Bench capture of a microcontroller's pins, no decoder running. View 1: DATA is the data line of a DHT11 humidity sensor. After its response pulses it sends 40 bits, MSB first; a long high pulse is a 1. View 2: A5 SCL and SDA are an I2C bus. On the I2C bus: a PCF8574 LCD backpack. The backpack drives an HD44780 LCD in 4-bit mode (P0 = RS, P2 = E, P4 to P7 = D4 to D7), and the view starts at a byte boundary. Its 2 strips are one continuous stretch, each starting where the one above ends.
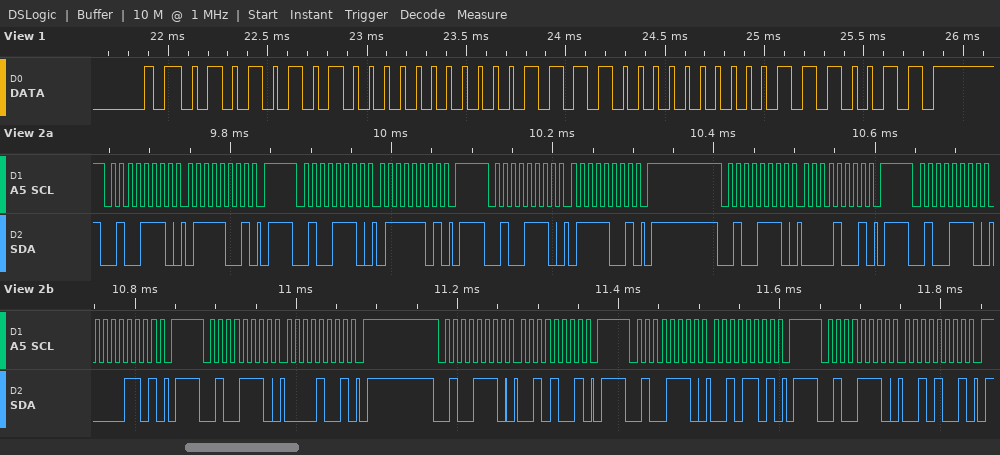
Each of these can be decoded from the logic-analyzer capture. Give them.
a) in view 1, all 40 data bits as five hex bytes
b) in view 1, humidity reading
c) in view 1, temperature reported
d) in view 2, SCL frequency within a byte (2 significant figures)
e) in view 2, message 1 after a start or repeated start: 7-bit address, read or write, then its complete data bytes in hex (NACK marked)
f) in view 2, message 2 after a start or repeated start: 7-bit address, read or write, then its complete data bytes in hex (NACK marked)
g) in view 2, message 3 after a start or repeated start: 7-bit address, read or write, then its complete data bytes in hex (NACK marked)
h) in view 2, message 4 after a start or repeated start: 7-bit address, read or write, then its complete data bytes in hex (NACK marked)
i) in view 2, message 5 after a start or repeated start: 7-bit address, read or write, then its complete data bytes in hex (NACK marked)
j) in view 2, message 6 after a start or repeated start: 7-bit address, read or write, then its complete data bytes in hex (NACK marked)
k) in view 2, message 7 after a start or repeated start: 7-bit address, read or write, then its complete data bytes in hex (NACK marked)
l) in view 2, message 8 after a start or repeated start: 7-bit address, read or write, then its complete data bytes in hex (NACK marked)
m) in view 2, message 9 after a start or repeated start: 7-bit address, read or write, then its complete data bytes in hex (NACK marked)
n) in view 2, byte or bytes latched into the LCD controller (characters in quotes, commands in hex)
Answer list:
55 00 1E 00 73
85 %
30.0 °C
100 kHz
0x27 write: 79
0x27 write: 7D
0x27 write: 79
0x27 write: 09
0x27 write: 0D
0x27 write: 09
0x27 write: 29
0x27 write: 2D
0x27 write: 29
'p'
